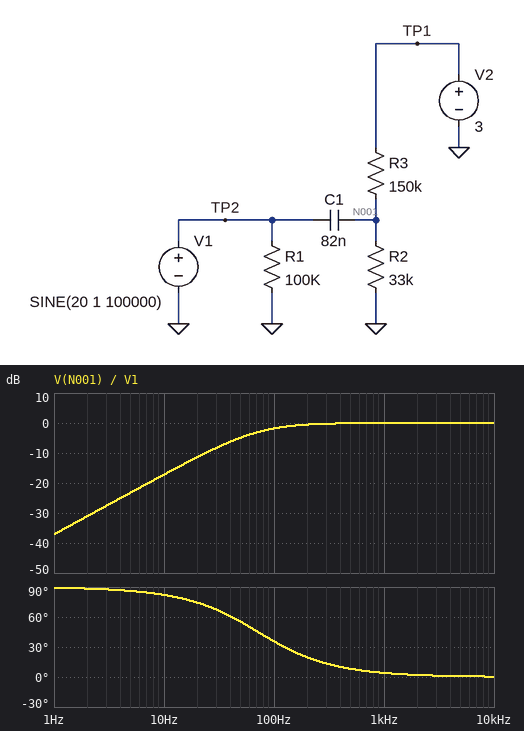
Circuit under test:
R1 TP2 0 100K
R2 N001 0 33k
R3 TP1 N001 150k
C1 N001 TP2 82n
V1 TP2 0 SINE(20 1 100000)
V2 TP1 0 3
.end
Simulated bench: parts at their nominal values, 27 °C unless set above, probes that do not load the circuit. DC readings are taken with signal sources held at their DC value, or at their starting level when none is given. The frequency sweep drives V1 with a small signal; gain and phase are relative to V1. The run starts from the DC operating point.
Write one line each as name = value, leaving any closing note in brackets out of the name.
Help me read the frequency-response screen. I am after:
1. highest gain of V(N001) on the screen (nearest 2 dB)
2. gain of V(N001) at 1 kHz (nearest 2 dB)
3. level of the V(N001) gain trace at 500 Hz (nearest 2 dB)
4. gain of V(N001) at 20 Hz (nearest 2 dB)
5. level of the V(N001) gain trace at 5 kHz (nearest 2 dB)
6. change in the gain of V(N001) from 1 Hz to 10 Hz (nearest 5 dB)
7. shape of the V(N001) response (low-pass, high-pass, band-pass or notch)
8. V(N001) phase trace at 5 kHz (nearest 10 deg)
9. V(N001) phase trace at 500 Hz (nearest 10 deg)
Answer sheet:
highest gain of V(N001) on the screen = 0 dB
gain of V(N001) at 1 kHz = 0 dB
level of the V(N001) gain trace at 500 Hz = 0 dB
gain of V(N001) at 20 Hz = -12 dB
level of the V(N001) gain trace at 5 kHz = 0 dB
change in the gain of V(N001) from 1 Hz to 10 Hz = 20 dB
shape of the V(N001) response = high-pass
V(N001) phase trace at 5 kHz = 0 deg
V(N001) phase trace at 500 Hz = 10 deg
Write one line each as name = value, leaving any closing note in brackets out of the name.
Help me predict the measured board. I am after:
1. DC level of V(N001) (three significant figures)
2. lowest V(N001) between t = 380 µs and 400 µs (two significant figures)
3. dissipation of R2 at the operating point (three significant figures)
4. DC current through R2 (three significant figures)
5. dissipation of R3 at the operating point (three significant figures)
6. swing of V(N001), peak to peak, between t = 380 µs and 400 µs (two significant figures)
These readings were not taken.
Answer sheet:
DC level of V(N001) = 541 mV
lowest V(N001) between t = 380 µs and 400 µs = -460 mV
dissipation of R2 at the operating point = 8.87 µW
DC current through R2 = 16.4 µA
dissipation of R3 at the operating point = 40.3 µW
swing of V(N001), peak to peak, between t = 380 µs and 400 µs = 2.0 V
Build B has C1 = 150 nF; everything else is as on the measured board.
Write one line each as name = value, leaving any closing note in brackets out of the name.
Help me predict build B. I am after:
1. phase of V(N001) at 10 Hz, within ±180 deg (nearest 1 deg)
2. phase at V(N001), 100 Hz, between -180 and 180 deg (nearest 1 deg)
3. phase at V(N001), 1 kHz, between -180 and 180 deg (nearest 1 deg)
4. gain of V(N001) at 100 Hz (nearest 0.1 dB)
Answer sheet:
phase of V(N001) at 10 Hz, within ±180 deg = 76 deg
phase at V(N001), 100 Hz, between -180 and 180 deg = 21 deg
phase at V(N001), 1 kHz, between -180 and 180 deg = 2 deg
gain of V(N001) at 100 Hz = -0.6 dB
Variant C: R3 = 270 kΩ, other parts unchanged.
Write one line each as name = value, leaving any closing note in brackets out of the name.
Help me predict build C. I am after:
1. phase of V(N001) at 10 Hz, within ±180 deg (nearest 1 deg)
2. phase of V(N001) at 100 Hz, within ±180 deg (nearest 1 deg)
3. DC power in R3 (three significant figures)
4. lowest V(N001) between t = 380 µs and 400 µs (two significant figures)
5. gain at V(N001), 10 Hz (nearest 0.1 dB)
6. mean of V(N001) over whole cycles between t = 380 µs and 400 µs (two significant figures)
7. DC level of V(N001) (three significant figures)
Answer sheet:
phase of V(N001) at 10 Hz, within ±180 deg = 81 deg
phase of V(N001) at 100 Hz, within ±180 deg = 33 deg
DC power in R3 = 26.5 µW
lowest V(N001) between t = 380 µs and 400 µs = -670 mV
gain at V(N001), 10 Hz = -16.5 dB
mean of V(N001) over whole cycles between t = 380 µs and 400 µs = 330 mV
DC level of V(N001) = 327 mV
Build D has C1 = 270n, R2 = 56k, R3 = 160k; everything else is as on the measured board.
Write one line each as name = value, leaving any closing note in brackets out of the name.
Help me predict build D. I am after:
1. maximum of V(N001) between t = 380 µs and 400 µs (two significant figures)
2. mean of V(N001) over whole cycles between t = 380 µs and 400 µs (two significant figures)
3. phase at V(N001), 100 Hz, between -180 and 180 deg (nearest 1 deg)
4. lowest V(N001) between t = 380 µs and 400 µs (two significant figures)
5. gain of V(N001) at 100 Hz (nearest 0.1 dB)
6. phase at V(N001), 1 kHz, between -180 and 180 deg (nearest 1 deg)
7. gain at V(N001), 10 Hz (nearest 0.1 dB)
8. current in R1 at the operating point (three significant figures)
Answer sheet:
maximum of V(N001) between t = 380 µs and 400 µs = 1.8 V
mean of V(N001) over whole cycles between t = 380 µs and 400 µs = 780 mV
phase at V(N001), 100 Hz, between -180 and 180 deg = 8 deg
lowest V(N001) between t = 380 µs and 400 µs = -220 mV
gain of V(N001) at 100 Hz = -0.1 dB
phase at V(N001), 1 kHz, between -180 and 180 deg = 1 deg
gain at V(N001), 10 Hz = -4.8 dB
current in R1 at the operating point = 200 µA
